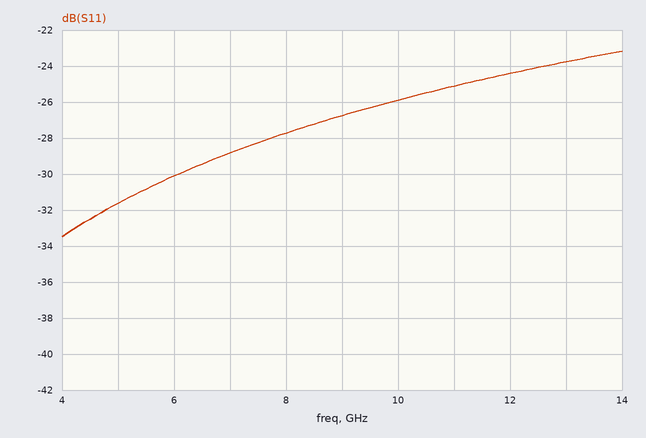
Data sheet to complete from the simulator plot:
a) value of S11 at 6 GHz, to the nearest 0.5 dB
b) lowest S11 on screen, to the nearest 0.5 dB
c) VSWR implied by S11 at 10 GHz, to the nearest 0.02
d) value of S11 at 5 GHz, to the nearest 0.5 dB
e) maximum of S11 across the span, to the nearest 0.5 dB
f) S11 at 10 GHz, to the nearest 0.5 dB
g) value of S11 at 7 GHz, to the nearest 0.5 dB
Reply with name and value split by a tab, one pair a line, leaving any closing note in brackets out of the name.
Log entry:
value of S11 at 6 GHz, to the nearest 0.5 dB	-30.0 dB
lowest S11 on screen, to the nearest 0.5 dB	-33.5 dB
VSWR implied by S11 at 10 GHz, to the nearest 0.02	1.10
value of S11 at 5 GHz, to the nearest 0.5 dB	-31.5 dB
maximum of S11 across the span, to the nearest 0.5 dB	-23.0 dB
S11 at 10 GHz, to the nearest 0.5 dB	-26.0 dB
value of S11 at 7 GHz, to the nearest 0.5 dB	-29.0 dB
